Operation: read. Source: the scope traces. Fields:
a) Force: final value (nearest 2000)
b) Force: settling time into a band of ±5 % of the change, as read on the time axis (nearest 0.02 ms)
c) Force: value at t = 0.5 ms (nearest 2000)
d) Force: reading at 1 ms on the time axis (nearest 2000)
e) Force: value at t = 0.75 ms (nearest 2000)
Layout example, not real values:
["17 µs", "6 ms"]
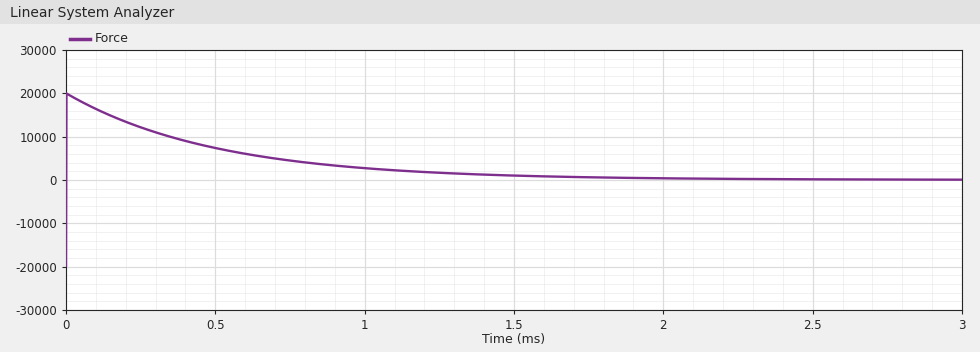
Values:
["0", "1.50 ms", "8000", "2000", "4000"]
